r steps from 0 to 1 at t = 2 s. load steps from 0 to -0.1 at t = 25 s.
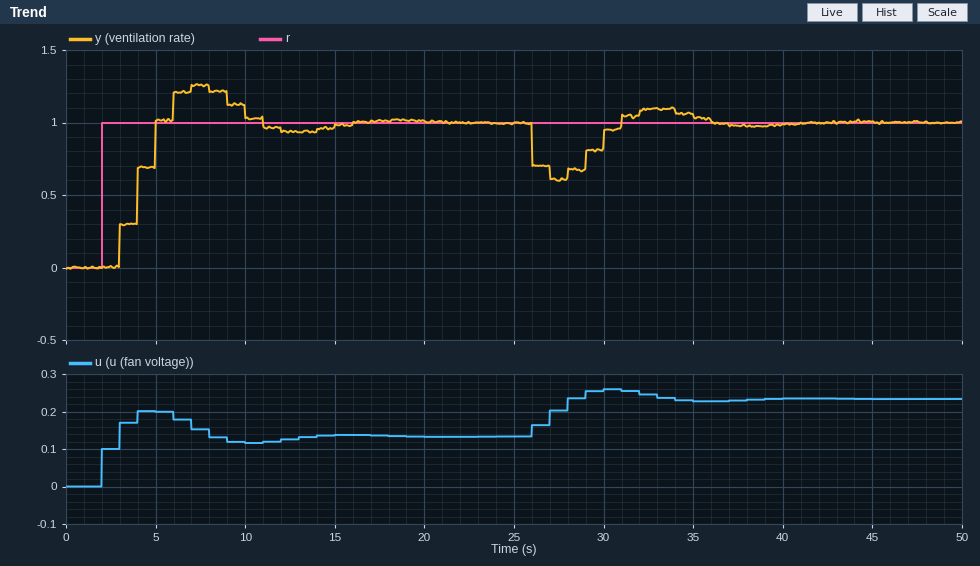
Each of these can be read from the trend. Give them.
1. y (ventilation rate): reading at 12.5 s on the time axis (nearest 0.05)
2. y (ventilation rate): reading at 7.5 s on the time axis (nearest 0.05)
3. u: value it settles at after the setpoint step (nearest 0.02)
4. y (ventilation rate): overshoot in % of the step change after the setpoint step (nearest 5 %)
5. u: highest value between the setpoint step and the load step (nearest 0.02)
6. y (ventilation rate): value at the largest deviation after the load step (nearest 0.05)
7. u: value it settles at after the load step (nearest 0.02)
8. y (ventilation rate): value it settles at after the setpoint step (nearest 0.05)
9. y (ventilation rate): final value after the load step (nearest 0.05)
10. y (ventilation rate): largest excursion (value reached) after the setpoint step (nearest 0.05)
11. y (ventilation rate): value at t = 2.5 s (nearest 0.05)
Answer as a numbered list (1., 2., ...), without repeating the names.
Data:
1. 0.95
2. 1.25
3. 0.14
4. 25 %
5. 0.20
6. 0.60
7. 0.24
8. 1.00
9. 1.00
10. 1.25
11. 0.00
